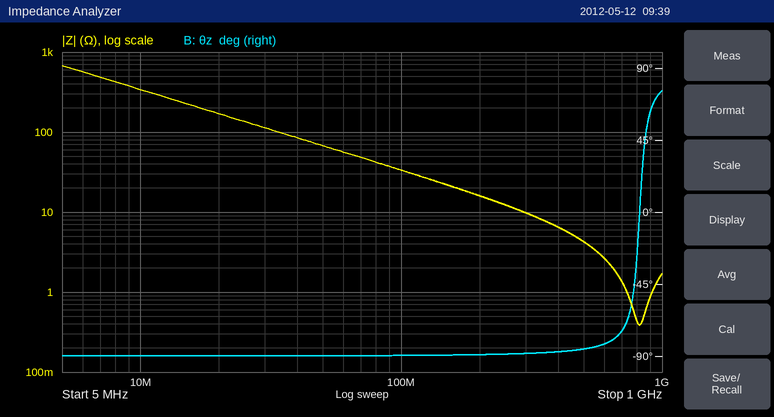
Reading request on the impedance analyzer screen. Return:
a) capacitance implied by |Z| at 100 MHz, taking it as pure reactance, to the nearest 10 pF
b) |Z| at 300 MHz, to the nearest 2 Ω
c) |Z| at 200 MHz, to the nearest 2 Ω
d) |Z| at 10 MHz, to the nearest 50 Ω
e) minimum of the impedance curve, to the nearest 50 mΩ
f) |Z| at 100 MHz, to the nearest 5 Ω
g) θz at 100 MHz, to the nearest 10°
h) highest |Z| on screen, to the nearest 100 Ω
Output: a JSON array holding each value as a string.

["50 pF", "10 Ω", "16 Ω", "350 Ω", "400 mΩ", "35 Ω", "-90°", "700 Ω"]
